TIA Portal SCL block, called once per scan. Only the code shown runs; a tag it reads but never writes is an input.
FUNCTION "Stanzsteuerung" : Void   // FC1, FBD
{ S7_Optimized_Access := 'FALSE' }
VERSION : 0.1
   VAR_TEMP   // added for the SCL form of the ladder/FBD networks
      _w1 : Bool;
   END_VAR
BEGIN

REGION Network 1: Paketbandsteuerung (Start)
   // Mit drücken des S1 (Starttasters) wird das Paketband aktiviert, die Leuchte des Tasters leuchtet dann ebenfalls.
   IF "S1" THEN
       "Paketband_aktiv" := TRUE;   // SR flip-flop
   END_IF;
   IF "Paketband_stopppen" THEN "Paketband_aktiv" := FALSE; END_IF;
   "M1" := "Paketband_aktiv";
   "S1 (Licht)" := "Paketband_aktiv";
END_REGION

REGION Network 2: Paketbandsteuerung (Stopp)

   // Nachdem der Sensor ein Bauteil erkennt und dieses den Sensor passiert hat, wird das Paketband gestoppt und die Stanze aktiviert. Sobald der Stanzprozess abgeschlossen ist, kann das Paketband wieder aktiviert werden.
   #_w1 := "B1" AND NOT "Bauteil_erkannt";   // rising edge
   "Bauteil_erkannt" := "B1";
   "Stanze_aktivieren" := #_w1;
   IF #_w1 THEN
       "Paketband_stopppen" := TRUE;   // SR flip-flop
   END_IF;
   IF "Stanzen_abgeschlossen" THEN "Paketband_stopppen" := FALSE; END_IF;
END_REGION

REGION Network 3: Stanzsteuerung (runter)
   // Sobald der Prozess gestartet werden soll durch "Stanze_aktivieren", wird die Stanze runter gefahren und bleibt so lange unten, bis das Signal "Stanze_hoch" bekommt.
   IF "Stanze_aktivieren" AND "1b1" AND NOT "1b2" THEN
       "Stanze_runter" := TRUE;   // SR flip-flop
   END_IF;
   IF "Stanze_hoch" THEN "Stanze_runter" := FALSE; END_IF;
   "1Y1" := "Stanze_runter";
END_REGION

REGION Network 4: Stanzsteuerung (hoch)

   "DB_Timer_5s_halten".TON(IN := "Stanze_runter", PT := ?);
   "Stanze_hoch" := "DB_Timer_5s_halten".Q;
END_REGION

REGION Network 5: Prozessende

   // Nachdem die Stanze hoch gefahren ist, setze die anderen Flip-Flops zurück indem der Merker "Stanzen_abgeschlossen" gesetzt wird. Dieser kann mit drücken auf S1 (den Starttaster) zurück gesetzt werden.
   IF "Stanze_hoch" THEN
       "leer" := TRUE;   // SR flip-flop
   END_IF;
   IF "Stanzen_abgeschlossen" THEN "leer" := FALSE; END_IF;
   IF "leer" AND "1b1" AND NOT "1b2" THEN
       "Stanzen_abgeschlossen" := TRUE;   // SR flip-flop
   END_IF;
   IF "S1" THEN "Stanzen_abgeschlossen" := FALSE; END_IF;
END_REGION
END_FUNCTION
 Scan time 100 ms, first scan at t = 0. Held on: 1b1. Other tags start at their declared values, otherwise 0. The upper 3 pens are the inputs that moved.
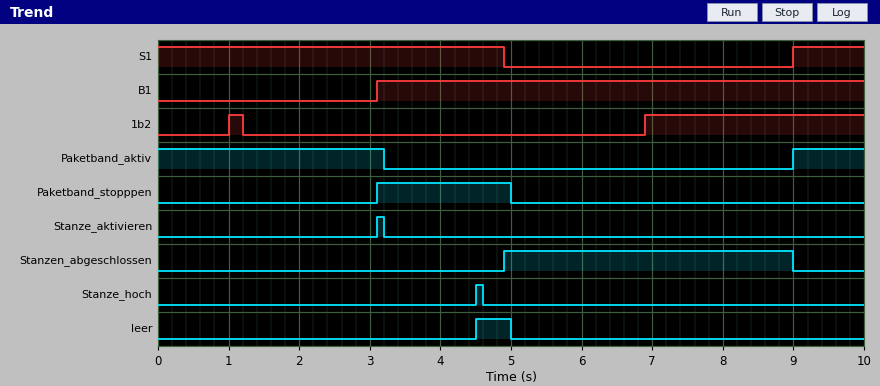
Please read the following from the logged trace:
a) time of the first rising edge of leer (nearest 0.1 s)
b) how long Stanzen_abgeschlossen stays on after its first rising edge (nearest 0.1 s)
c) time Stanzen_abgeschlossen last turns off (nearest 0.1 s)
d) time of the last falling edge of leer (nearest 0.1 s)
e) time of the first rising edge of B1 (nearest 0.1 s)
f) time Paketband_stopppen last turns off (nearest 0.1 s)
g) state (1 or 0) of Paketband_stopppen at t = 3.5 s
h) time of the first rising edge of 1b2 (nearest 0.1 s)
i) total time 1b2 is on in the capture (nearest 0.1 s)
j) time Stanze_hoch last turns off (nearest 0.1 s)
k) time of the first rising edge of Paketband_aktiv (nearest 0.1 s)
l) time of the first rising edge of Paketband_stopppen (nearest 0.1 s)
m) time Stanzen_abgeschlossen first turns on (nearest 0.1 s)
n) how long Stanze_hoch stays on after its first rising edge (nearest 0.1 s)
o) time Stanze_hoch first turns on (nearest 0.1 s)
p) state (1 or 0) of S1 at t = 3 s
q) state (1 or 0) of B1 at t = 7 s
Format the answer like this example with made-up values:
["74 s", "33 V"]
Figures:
["4.5 s", "4.1 s", "9.0 s", "5.0 s", "3.1 s", "5.0 s", "1", "1.0 s", "3.3 s", "4.6 s", "9.0 s", "3.1 s", "4.9 s", "0.1 s", "4.5 s", "1", "1"]
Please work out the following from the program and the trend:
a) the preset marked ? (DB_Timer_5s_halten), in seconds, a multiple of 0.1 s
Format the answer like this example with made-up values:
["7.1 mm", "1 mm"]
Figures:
["1.4 s"]
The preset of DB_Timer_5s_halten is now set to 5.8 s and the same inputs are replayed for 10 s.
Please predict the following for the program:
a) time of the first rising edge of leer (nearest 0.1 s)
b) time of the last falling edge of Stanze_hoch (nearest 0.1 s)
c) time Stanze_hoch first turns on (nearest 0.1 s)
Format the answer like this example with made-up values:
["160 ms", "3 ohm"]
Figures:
["8.9 s", "9.0 s", "8.9 s"]
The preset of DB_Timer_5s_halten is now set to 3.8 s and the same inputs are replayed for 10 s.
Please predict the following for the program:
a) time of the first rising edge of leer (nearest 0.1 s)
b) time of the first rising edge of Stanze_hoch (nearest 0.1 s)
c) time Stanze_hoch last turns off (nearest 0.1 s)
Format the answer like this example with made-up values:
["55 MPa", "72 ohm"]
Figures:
["6.9 s", "6.9 s", "7.0 s"]
